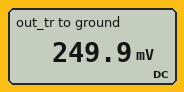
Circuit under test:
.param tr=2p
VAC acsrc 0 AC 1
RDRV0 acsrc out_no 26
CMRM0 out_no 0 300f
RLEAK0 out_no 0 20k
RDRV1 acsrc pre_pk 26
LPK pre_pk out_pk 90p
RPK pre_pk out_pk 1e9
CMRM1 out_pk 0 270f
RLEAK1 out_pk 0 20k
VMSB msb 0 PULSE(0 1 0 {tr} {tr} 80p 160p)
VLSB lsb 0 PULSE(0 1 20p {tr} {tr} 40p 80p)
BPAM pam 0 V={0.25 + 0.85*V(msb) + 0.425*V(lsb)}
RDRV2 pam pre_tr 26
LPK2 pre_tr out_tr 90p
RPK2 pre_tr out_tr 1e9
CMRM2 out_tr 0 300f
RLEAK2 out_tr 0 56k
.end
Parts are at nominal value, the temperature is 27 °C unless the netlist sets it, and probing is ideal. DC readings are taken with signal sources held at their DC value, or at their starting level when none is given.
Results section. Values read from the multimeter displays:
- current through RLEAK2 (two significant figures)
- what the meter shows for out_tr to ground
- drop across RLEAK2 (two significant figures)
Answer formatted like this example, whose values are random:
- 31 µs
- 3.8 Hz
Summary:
- 4.5 µA
- 249.9 mV
- 250 mV
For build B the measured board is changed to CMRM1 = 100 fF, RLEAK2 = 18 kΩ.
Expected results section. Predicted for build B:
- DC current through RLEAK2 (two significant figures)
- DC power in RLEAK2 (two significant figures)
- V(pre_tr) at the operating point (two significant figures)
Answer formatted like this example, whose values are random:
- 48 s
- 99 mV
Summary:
- 14 µA
- 3.5 µW
- 250 mV
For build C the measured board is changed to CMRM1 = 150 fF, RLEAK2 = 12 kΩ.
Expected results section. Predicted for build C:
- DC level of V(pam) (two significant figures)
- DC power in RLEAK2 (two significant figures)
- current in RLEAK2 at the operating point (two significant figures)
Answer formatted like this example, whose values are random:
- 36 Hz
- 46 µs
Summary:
- 250 mV
- 5.2 µW
- 21 µA
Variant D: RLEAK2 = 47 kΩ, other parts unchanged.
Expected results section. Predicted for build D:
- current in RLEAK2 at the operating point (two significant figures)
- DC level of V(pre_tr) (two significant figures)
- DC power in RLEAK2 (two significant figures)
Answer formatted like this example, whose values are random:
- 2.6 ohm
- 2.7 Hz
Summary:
- 5.3 µA
- 250 mV
- 1.3 µW
